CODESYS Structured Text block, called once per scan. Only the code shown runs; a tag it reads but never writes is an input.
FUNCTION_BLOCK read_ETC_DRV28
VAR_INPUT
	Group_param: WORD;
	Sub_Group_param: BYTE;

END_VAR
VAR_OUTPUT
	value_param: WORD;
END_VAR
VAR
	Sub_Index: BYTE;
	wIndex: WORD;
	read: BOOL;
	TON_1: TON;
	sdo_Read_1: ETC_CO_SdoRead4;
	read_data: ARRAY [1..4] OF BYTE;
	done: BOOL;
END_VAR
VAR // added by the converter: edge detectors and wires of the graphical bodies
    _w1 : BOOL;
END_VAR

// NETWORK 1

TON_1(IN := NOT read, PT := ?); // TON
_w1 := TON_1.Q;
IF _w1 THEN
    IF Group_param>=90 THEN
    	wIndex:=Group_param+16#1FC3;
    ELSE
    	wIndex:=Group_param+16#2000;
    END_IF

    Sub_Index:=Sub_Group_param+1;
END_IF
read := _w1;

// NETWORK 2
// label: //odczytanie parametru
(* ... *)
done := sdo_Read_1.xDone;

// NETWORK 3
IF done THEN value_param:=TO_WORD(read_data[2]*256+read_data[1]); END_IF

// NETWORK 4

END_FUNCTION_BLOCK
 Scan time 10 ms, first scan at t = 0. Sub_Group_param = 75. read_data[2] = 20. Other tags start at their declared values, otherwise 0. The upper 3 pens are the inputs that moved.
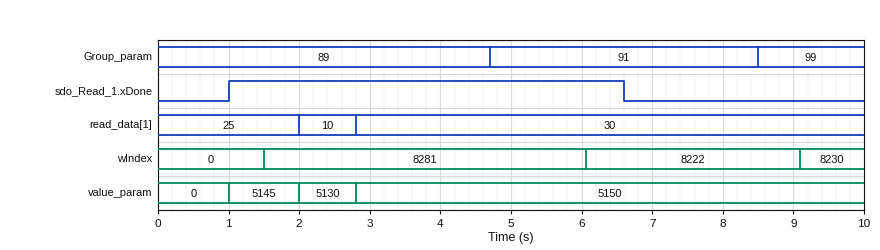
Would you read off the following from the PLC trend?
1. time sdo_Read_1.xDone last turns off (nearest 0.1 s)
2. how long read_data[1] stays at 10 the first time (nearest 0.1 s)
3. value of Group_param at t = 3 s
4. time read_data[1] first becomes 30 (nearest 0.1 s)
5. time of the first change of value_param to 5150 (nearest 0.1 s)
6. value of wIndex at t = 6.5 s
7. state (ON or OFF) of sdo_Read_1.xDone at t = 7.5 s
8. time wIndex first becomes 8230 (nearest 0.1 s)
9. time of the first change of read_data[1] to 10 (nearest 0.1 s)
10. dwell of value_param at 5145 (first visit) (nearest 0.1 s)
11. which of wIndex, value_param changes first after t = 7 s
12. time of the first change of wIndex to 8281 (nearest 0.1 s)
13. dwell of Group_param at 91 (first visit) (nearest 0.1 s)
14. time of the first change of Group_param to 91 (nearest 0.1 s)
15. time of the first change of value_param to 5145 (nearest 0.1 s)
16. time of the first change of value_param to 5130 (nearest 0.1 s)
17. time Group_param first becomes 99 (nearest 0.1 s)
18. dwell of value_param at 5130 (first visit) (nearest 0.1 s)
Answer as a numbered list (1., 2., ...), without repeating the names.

1. 6.6 s
2. 0.8 s
3. 89
4. 2.8 s
5. 2.8 s
6. 8222
7. OFF
8. 9.1 s
9. 2.0 s
10. 1.0 s
11. wIndex
12. 1.5 s
13. 3.8 s
14. 4.7 s
15. 1.0 s
16. 2.0 s
17. 8.5 s
18. 0.8 s
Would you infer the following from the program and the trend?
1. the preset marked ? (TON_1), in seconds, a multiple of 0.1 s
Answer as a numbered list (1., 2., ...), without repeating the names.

1. 1.5 s
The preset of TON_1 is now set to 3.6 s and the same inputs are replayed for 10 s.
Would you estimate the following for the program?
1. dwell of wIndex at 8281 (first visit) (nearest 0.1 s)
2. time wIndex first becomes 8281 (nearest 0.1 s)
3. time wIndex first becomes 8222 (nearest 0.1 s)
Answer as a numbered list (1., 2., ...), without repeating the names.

1. 3.6 s
2. 3.6 s
3. 7.2 s
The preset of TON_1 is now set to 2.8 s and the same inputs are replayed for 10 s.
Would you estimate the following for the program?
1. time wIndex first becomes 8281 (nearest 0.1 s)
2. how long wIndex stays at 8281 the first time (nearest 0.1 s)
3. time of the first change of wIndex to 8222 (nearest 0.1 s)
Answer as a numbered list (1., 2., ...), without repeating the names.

1. 2.8 s
2. 2.8 s
3. 5.6 s
